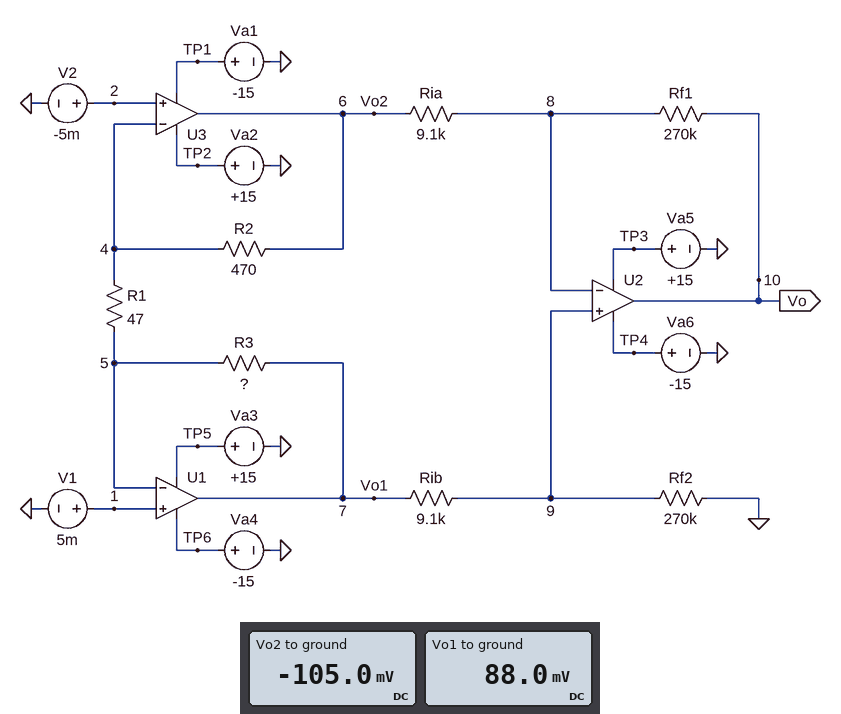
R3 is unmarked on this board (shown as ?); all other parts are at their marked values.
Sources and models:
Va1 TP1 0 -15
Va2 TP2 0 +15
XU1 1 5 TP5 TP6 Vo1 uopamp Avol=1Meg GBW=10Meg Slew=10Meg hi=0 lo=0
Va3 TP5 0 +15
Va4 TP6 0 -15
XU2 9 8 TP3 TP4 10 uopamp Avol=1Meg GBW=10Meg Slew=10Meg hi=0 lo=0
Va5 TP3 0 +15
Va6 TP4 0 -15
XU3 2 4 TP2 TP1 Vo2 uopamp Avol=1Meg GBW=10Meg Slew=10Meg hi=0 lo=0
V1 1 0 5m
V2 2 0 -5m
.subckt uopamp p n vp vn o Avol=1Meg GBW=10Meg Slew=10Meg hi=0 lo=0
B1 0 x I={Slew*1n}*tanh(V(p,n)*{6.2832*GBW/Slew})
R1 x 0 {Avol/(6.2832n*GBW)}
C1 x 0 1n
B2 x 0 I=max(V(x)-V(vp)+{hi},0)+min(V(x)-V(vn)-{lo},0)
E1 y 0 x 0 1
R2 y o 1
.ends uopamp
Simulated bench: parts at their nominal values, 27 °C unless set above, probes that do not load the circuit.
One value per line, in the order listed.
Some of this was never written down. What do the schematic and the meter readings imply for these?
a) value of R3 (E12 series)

390 Ω
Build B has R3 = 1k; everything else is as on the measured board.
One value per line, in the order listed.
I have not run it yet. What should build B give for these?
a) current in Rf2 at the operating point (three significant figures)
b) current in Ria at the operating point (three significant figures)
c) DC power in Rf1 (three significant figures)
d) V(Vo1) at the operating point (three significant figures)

780 nA
34.7 µA
325 µW
218 mV
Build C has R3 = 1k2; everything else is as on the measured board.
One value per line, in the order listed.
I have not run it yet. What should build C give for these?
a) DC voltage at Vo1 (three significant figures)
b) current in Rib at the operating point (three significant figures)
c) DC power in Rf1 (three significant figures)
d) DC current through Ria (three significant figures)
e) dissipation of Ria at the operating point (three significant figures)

260 mV
933 nA
415 µW
39.2 µA
14.0 µW
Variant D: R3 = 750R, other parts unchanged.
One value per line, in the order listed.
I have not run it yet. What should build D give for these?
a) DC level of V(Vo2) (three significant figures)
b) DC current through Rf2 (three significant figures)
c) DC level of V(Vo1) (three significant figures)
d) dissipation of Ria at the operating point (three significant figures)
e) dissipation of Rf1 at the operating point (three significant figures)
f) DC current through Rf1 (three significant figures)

-105 mV
590 nA
165 mV
7.67 µW
228 µW
29.0 µA
